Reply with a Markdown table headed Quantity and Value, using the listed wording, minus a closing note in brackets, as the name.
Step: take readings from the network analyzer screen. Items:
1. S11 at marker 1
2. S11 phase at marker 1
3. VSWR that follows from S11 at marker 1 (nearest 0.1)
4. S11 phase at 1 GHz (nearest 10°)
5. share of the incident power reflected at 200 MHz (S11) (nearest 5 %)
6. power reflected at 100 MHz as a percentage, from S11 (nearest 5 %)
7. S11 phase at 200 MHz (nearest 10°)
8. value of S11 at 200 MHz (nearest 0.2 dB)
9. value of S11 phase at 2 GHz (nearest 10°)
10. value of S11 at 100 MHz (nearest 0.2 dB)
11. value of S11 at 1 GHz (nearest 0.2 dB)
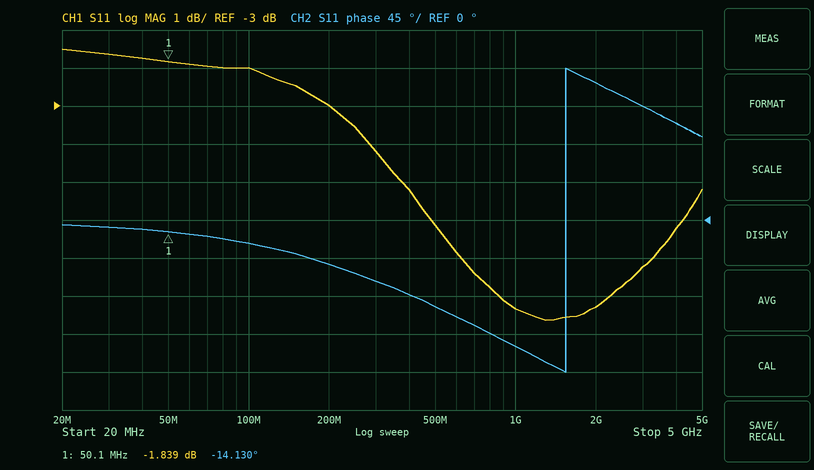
| Quantity | Value |
|---|---|
| S11 at marker 1 | -1.839 dB |
| S11 phase at marker 1 | -14.130° |
| VSWR that follows from S11 at marker 1 | 9.5 |
| S11 phase at 1 GHz | -150° |
| share of the incident power reflected at 200 MHz (S11) | 50 % |
| power reflected at 100 MHz as a percentage, from S11 | 65 % |
| S11 phase at 200 MHz | -50° |
| value of S11 at 200 MHz | -3.0 dB |
| value of S11 phase at 2 GHz | 160° |
| value of S11 at 100 MHz | -2.0 dB |
| value of S11 at 1 GHz | -8.4 dB |
